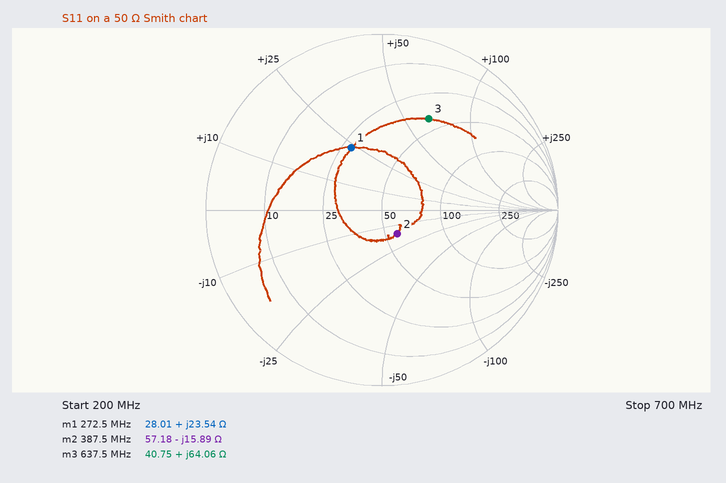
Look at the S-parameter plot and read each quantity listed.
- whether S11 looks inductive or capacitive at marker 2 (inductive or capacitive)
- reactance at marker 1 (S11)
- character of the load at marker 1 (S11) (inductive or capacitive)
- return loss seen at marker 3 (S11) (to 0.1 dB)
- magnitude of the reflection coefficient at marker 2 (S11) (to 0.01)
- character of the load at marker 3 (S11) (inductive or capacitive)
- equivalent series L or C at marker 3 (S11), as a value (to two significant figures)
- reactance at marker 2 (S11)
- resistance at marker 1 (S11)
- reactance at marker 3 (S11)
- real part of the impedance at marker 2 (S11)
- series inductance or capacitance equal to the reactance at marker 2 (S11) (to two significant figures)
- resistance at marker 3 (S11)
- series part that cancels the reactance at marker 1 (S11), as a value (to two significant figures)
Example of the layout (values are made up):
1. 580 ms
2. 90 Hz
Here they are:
1. capacitive
2. +23.54 Ω
3. inductive
4. 4.7 dB
5. 0.16
6. inductive
7. 16 nH
8. -15.89 Ω
9. 28.01 Ω
10. +64.06 Ω
11. 57.18 Ω
12. 26 pF
13. 40.75 Ω
14. 25 pF
